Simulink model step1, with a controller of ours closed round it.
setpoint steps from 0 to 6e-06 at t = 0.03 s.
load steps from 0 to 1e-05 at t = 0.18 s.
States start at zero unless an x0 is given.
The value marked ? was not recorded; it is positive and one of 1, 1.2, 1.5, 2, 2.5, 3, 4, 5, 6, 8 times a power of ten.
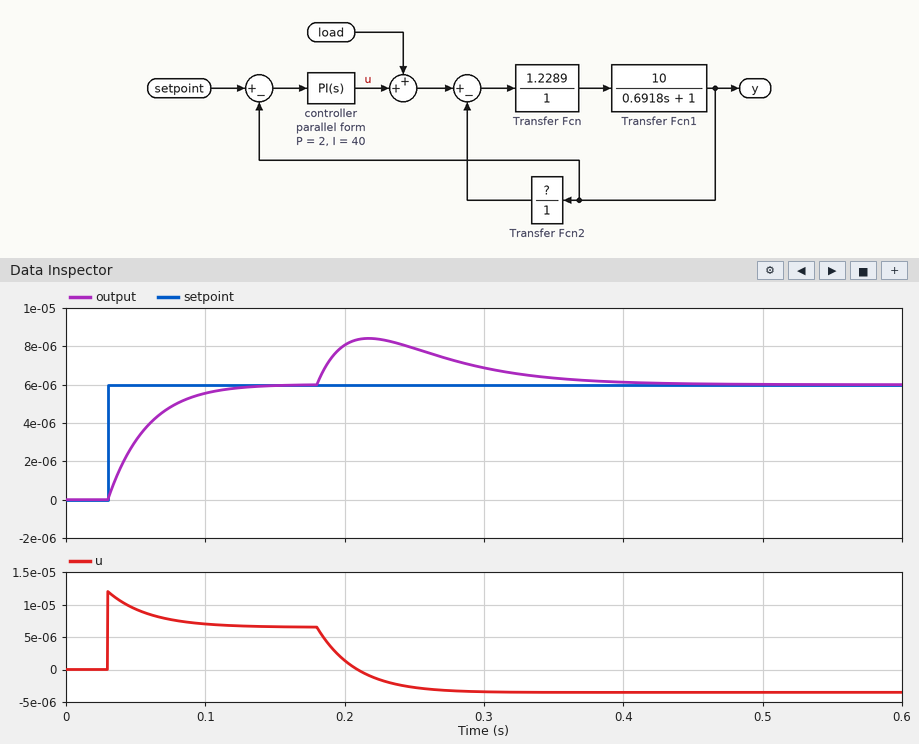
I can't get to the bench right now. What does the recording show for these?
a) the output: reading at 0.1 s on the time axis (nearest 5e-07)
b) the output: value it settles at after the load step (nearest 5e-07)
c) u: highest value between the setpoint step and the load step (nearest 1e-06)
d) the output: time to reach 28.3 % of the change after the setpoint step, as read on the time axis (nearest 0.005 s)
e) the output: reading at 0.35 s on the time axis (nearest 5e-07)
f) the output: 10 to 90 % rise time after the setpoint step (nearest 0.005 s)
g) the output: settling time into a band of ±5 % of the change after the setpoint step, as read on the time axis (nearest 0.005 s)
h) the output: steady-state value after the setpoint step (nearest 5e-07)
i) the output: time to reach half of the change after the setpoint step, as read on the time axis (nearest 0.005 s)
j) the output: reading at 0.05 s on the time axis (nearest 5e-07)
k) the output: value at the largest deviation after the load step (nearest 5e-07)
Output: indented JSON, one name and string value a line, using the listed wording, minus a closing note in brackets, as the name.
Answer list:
{
  "the output: reading at 0.1 s on the time axis": "0.0000055",
  "the output: value it settles at after the load step": "0.0000060",
  "u: highest value between the setpoint step and the load step": "0.000012",
  "the output: time to reach 28.3 % of the change after the setpoint step, as read on the time axis": "0.040 s",
  "the output: reading at 0.35 s on the time axis": "0.0000065",
  "the output: 10 to 90 % rise time after the setpoint step": "0.060 s",
  "the output: settling time into a band of ±5 % of the change after the setpoint step, as read on the time axis": "0.110 s",
  "the output: steady-state value after the setpoint step": "0.0000060",
  "the output: time to reach half of the change after the setpoint step, as read on the time axis": "0.050 s",
  "the output: reading at 0.05 s on the time axis": "0.0000030",
  "the output: value at the largest deviation after the load step": "0.0000085"
}
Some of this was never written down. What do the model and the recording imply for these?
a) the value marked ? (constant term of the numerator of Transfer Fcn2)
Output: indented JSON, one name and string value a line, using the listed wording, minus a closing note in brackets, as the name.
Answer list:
{
  "the value marked ?": "1"
}
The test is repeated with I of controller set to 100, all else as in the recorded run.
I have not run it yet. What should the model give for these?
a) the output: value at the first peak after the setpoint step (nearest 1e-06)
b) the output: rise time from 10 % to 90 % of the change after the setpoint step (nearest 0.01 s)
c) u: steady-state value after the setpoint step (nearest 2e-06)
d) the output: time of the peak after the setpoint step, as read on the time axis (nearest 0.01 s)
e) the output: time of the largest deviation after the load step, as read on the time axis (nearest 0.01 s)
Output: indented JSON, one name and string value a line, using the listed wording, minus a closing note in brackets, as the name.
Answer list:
{
  "the output: value at the first peak after the setpoint step": "0.000007",
  "the output: rise time from 10 % to 90 % of the change after the setpoint step": "0.03 s",
  "u: steady-state value after the setpoint step": "0.000006",
  "the output: time of the peak after the setpoint step, as read on the time axis": "0.10 s",
  "the output: time of the largest deviation after the load step, as read on the time axis": "0.21 s"
}
